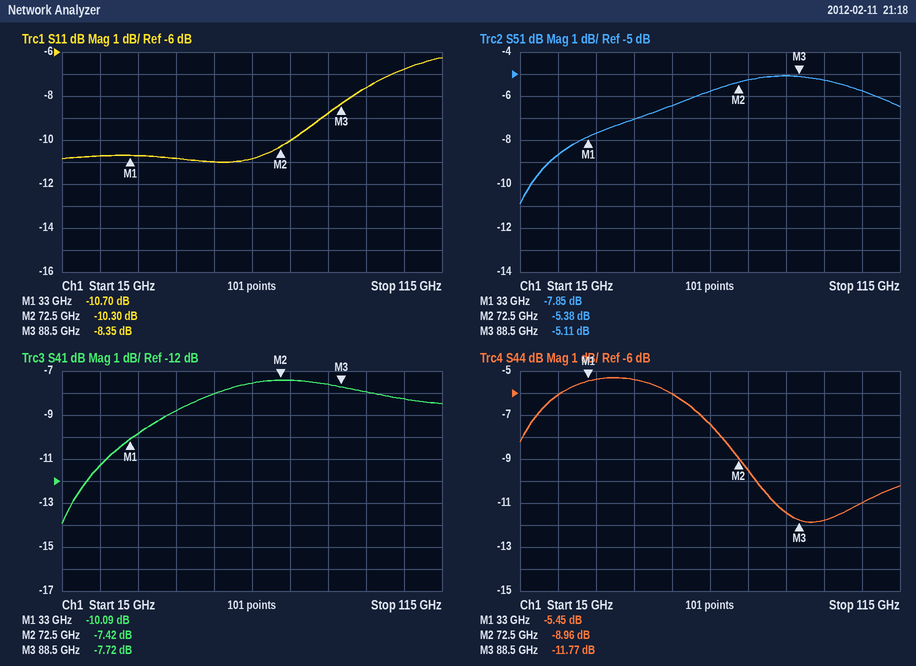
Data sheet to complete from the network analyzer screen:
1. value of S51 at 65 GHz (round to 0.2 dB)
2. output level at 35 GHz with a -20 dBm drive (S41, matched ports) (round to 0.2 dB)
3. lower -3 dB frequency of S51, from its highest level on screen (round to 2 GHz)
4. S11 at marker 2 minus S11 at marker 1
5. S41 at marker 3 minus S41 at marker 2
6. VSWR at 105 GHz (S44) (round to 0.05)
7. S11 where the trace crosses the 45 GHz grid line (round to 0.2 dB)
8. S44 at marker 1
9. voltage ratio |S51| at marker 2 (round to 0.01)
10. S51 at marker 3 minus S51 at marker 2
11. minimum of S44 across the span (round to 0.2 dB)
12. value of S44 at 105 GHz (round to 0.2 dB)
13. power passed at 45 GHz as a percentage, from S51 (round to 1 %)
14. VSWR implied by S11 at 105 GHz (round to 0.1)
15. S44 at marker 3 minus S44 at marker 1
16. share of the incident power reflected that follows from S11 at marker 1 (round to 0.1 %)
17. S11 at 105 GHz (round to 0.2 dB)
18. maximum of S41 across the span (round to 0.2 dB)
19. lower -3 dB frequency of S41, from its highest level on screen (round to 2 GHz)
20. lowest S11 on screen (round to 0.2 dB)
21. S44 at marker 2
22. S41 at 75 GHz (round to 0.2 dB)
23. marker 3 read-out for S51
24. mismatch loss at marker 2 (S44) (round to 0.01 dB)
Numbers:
-5.8 dB
-29.8 dBm
30 GHz
0.40 dB
-0.30 dB
1.80
-10.8 dB
-5.45 dB
0.54
0.27 dB
-11.8 dB
-11.0 dB
20 %
2.7
-6.32 dB
8.5 %
-6.8 dB
-7.4 dB
30 GHz
-11.0 dB
-8.96 dB
-7.4 dB
-5.11 dB
0.59 dB
